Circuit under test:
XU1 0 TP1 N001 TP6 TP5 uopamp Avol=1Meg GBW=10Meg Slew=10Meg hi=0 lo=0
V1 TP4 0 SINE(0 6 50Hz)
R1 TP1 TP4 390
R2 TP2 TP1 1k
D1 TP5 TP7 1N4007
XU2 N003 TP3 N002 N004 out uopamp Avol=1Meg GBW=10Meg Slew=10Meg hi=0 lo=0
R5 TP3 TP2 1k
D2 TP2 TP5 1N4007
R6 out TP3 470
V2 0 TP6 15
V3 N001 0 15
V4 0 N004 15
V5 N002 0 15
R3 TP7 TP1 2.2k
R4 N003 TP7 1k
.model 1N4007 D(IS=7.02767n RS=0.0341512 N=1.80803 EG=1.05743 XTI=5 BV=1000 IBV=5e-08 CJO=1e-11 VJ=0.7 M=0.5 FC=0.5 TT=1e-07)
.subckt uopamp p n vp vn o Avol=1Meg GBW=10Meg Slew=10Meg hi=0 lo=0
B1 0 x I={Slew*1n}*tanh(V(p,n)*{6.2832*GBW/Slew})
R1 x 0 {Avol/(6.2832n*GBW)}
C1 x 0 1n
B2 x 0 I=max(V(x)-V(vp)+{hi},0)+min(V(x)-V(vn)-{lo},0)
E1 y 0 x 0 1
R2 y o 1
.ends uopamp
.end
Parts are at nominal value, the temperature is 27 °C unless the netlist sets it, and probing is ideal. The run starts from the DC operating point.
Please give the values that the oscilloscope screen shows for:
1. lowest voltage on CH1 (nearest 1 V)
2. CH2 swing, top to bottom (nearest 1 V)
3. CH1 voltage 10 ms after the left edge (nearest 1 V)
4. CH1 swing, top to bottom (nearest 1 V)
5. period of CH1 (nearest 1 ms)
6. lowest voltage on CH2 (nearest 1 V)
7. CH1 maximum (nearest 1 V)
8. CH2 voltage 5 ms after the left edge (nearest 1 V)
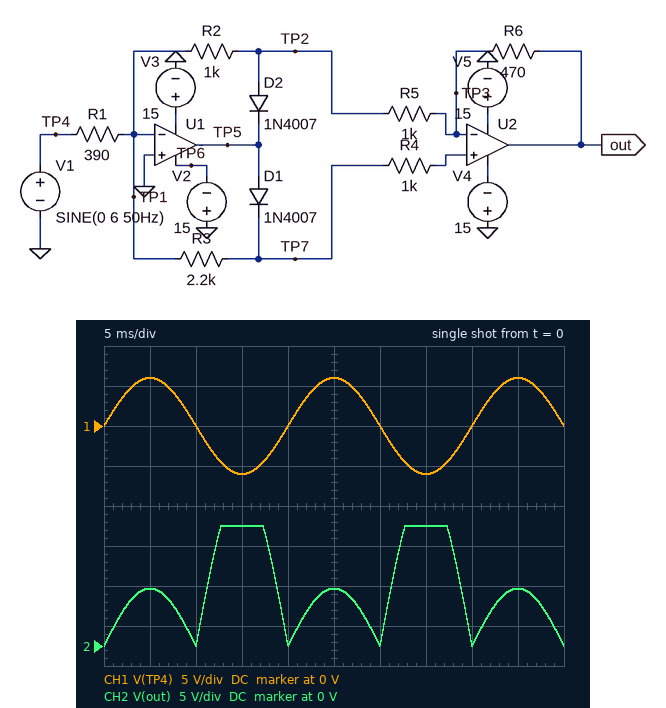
-6 V
15 V
0 V
12 V
20 ms
0 V
6 V
7 V
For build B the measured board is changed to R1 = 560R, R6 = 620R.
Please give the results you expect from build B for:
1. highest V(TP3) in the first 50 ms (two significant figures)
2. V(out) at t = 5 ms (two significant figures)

11 V
6.6 V
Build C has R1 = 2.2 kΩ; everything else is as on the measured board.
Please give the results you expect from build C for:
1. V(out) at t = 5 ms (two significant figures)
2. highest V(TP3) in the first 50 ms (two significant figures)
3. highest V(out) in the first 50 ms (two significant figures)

1.3 V
2.9 V
3.5 V
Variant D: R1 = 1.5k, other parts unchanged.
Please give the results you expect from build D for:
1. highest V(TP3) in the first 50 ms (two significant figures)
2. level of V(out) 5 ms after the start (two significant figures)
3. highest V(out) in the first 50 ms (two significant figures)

4.2 V
1.9 V
5.2 V
